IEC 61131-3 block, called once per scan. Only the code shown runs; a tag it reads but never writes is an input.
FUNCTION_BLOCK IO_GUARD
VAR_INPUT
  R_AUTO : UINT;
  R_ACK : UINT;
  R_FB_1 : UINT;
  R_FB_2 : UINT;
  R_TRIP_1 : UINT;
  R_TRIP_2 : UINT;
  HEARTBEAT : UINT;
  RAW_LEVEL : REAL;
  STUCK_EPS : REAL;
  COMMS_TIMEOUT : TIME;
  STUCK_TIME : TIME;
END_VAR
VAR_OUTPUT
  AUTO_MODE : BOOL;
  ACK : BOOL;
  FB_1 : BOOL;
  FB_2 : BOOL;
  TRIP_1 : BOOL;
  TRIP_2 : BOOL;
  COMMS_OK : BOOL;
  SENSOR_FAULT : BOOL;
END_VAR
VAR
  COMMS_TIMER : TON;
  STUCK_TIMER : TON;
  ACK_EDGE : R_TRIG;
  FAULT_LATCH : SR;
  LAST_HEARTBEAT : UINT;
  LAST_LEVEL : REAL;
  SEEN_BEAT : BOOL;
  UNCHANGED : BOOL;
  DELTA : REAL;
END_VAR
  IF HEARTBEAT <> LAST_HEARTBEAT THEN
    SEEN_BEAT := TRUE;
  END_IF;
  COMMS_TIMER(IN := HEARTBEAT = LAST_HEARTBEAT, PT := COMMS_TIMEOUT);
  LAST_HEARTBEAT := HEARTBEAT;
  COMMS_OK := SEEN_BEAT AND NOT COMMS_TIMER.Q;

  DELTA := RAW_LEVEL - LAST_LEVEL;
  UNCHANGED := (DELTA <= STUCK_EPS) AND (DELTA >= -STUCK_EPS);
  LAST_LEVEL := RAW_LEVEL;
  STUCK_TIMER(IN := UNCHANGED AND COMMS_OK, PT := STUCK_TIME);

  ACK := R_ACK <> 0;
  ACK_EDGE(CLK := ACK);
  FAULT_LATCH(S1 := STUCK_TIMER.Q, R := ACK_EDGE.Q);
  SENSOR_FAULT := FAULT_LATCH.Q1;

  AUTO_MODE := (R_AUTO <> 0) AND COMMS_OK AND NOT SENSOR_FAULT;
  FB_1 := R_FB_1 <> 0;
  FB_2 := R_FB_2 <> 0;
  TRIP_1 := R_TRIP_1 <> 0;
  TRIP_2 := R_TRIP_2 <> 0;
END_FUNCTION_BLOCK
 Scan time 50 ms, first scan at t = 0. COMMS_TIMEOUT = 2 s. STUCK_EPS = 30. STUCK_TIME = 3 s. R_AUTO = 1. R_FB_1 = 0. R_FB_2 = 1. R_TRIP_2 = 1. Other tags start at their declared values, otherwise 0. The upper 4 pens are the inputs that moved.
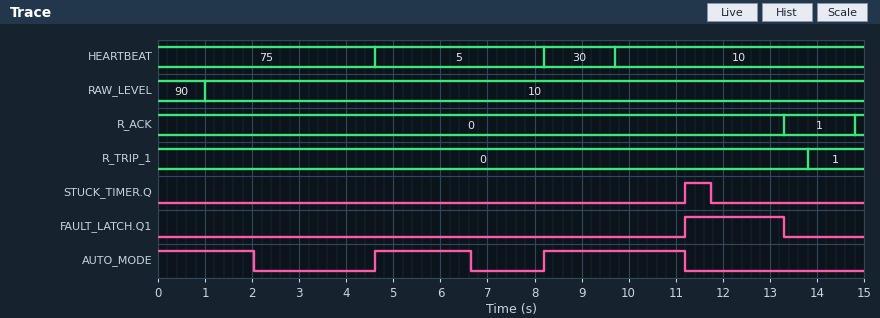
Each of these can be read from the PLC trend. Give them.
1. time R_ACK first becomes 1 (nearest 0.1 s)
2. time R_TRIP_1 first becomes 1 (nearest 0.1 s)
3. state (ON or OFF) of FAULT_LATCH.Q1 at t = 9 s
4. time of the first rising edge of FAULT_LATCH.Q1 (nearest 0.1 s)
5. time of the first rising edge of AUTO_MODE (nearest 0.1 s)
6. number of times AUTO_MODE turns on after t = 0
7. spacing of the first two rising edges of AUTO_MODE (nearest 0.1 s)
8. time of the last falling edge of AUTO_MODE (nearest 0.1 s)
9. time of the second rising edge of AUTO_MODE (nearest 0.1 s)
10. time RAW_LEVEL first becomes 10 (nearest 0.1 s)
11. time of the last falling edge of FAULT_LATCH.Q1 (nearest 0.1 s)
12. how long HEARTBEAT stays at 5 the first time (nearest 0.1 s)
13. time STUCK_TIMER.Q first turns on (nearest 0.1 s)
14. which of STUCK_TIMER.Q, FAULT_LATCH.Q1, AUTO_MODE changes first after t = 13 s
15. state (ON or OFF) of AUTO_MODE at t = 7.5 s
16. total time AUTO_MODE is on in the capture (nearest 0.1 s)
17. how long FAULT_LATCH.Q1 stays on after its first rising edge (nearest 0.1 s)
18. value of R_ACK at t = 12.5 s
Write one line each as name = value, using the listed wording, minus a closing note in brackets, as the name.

time R_ACK first becomes 1 = 13.3 s
time R_TRIP_1 first becomes 1 = 13.8 s
state (ON or OFF) of FAULT_LATCH.Q1 at t = 9 s = OFF
time of the first rising edge of FAULT_LATCH.Q1 = 11.2 s
time of the first rising edge of AUTO_MODE = 4.6 s
number of times AUTO_MODE turns on after t = 0 = 2
spacing of the first two rising edges of AUTO_MODE = 3.6 s
time of the last falling edge of AUTO_MODE = 11.2 s
time of the second rising edge of AUTO_MODE = 8.2 s
time RAW_LEVEL first becomes 10 = 1.0 s
time of the last falling edge of FAULT_LATCH.Q1 = 13.3 s
how long HEARTBEAT stays at 5 the first time = 3.6 s
time STUCK_TIMER.Q first turns on = 11.2 s
which of STUCK_TIMER.Q, FAULT_LATCH.Q1, AUTO_MODE changes first after t = 13 s = FAULT_LATCH.Q1
state (ON or OFF) of AUTO_MODE at t = 7.5 s = OFF
total time AUTO_MODE is on in the capture = 7.1 s
how long FAULT_LATCH.Q1 stays on after its first rising edge = 2.1 s
value of R_ACK at t = 12.5 s = 0
